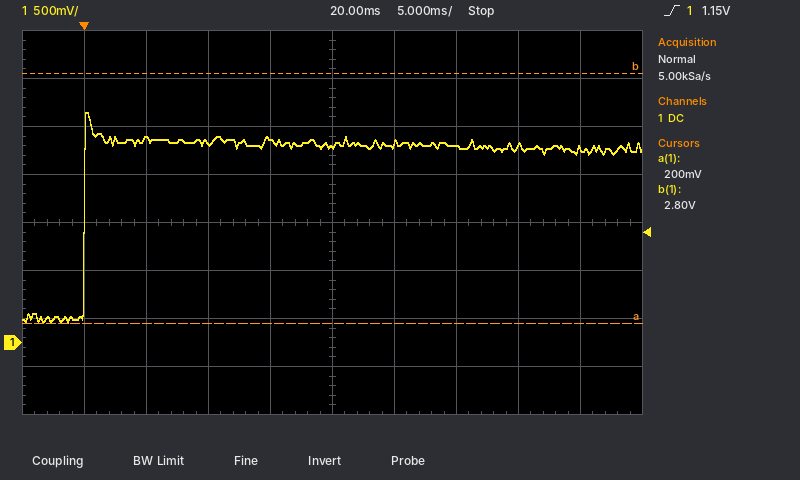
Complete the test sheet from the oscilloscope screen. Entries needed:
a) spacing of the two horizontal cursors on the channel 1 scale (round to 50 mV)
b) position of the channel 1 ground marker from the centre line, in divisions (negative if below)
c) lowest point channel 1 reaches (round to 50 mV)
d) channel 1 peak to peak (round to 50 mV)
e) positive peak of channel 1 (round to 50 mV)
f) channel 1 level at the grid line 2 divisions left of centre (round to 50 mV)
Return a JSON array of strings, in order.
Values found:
["2.60 V", "-2.5 div", "200 mV", "2.20 V", "2.40 V", "2.10 V"]
